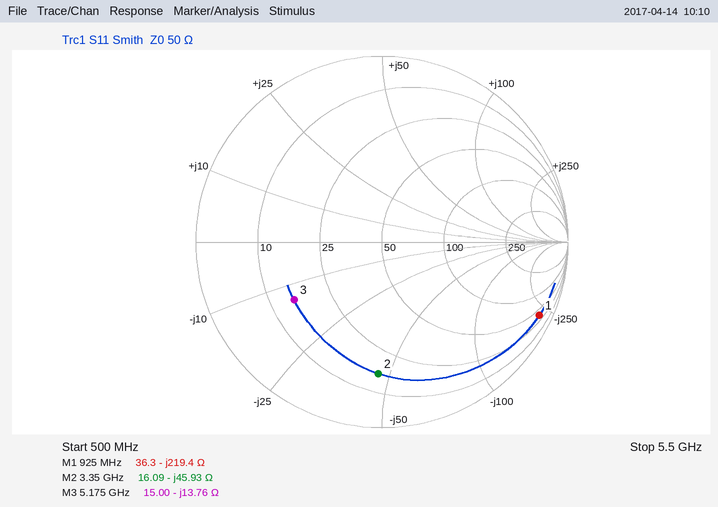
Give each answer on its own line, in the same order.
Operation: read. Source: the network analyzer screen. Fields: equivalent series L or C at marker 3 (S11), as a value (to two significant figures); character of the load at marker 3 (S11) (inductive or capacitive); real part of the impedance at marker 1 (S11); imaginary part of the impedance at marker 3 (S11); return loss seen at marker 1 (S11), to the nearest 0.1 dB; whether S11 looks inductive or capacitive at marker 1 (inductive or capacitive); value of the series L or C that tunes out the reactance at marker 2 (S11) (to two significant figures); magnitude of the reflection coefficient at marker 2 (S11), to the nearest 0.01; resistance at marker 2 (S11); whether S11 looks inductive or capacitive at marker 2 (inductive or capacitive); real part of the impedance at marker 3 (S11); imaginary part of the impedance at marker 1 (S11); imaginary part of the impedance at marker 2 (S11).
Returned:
2.2 pF
capacitive
36.3 Ω
-13.76 Ω
0.6 dB
capacitive
2.2 nH
0.71
16.09 Ω
capacitive
15.00 Ω
-219.4 Ω
-45.93 Ω
